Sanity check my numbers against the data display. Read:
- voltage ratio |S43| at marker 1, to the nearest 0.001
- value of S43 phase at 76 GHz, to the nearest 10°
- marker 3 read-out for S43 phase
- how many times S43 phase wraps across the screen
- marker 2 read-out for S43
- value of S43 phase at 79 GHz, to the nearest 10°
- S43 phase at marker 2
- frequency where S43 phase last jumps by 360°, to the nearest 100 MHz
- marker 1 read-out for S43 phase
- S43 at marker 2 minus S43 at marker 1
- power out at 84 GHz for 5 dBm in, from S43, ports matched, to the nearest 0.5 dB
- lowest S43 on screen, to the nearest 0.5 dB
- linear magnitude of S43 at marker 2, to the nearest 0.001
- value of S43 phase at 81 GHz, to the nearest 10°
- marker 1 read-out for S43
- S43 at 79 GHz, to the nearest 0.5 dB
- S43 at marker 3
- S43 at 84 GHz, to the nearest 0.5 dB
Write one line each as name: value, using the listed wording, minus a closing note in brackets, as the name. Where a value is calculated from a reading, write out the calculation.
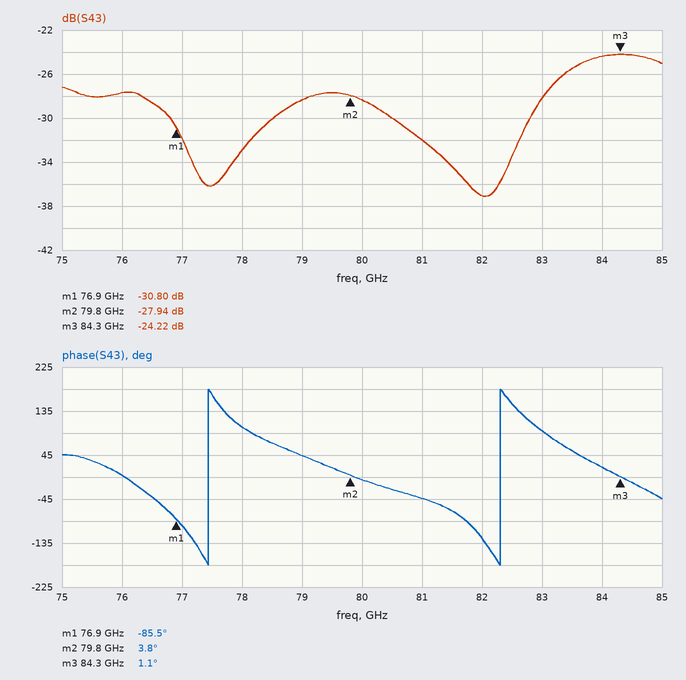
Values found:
voltage ratio |S43| at marker 1, to the nearest 0.001: 10^(-30.8/20) ≈ 0.029
value of S43 phase at 76 GHz, to the nearest 10°: 0°
marker 3 read-out for S43 phase: 1.1°
how many times S43 phase wraps across the screen: 2
marker 2 read-out for S43: -27.94 dB
value of S43 phase at 79 GHz, to the nearest 10°: 40°
S43 phase at marker 2: 3.8°
frequency where S43 phase last jumps by 360°, to the nearest 100 MHz: 82.3 GHz
marker 1 read-out for S43 phase: -85.5°
S43 at marker 2 minus S43 at marker 1: -27.94 − (-30.8) = 2.86 dB
power out at 84 GHz for 5 dBm in, from S43, ports matched, to the nearest 0.5 dB: 5 dBm + (-24.5 dB) = -19.5 dBm
lowest S43 on screen, to the nearest 0.5 dB: -37.0 dB
linear magnitude of S43 at marker 2, to the nearest 0.001: 10^(-27.94/20) ≈ 0.040
value of S43 phase at 81 GHz, to the nearest 10°: -40°
marker 1 read-out for S43: -30.80 dB
S43 at 79 GHz, to the nearest 0.5 dB: -28.5 dB
S43 at marker 3: -24.22 dB
S43 at 84 GHz, to the nearest 0.5 dB: -24.5 dB
